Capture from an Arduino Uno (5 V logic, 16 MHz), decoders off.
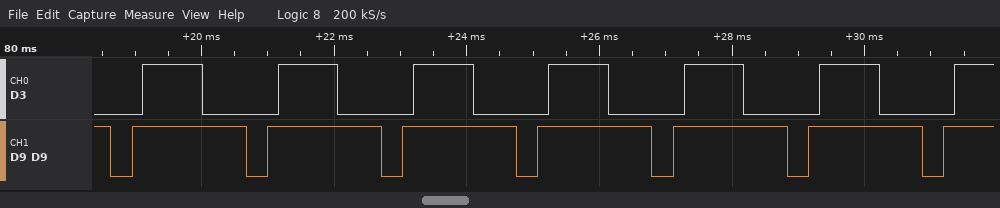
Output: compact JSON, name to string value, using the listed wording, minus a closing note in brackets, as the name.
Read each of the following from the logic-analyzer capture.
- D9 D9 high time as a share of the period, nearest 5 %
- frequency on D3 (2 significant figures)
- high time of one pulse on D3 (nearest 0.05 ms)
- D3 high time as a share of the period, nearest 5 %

{"D9 D9 high time as a share of the period, nearest 5 %": "85 %", "frequency on D3": "490 Hz", "high time of one pulse on D3": "0.90 ms", "D3 high time as a share of the period, nearest 5 %": "45 %"}
